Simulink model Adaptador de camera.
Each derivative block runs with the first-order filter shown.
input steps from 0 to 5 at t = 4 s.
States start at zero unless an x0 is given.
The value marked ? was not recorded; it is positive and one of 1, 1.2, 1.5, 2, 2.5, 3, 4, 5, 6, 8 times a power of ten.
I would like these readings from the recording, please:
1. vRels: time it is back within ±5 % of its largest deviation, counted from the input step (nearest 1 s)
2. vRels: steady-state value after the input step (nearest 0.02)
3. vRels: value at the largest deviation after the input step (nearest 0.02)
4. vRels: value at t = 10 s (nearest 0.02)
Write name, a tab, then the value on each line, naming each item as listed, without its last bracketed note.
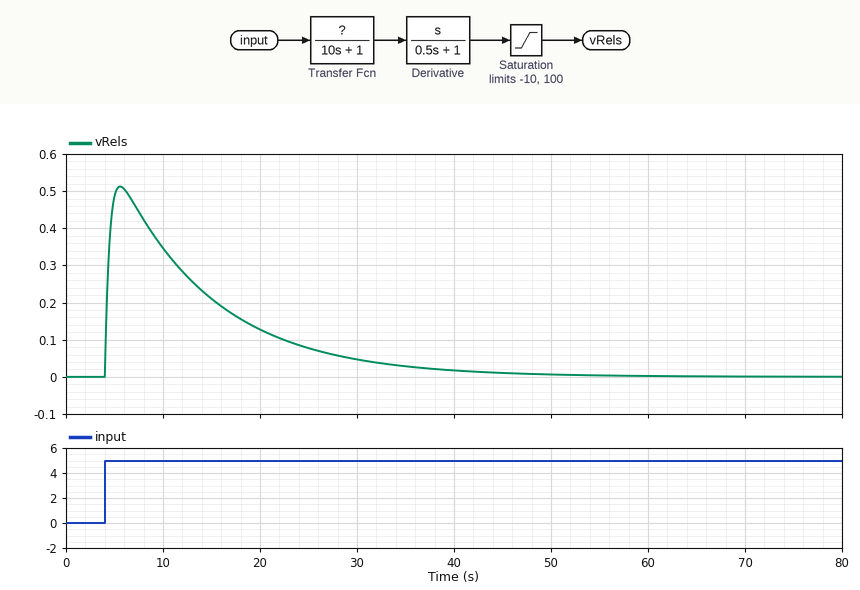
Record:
vRels: time it is back within ±5 % of its largest deviation, counted from the input step	32 s
vRels: steady-state value after the input step	0.00
vRels: value at the largest deviation after the input step	0.52
vRels: value at t = 10 s	0.34
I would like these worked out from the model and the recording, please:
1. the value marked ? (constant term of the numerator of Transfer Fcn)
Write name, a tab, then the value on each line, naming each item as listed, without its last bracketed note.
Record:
the value marked ?	1.2
